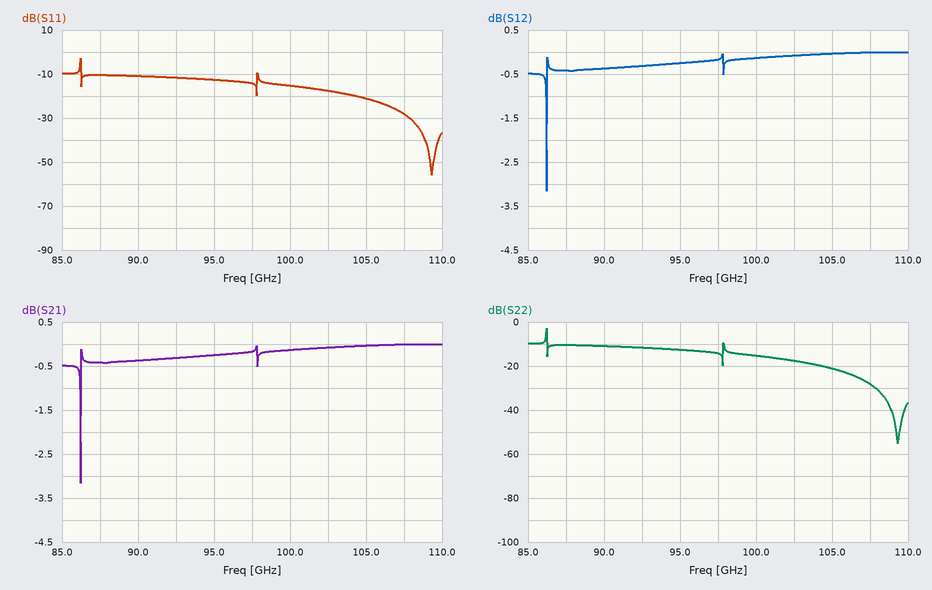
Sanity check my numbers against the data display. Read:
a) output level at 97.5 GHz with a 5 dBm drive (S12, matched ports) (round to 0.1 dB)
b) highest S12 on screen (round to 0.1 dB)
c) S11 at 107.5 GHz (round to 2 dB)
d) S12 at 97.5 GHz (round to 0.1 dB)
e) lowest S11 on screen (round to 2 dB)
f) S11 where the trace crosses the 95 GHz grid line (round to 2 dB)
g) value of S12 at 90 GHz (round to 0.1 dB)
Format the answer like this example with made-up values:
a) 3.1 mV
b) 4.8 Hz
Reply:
a) 4.8 dBm
b) 0.0 dB
c) -28 dB
d) -0.2 dB
e) -56 dB
f) -12 dB
g) -0.4 dB
